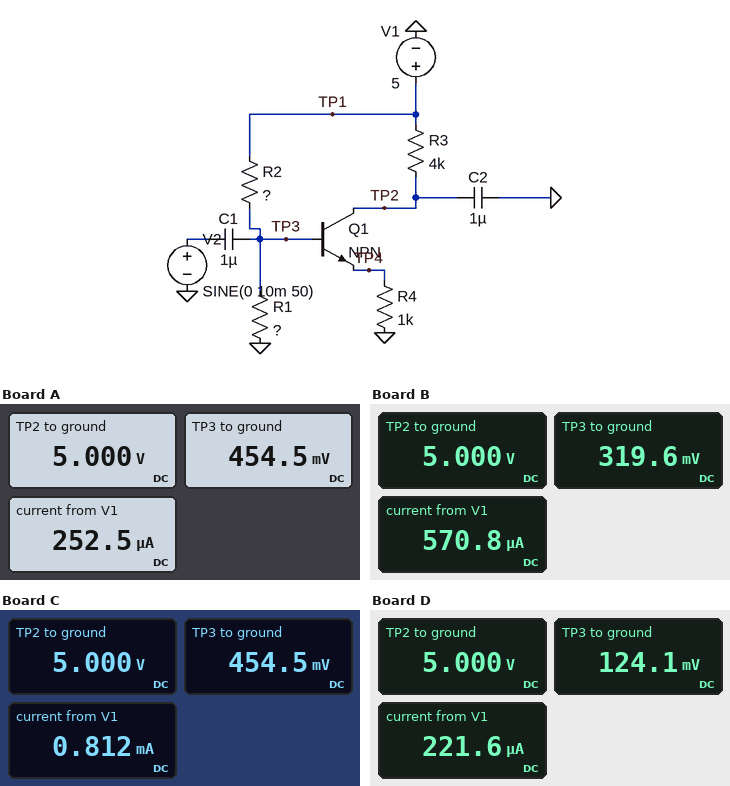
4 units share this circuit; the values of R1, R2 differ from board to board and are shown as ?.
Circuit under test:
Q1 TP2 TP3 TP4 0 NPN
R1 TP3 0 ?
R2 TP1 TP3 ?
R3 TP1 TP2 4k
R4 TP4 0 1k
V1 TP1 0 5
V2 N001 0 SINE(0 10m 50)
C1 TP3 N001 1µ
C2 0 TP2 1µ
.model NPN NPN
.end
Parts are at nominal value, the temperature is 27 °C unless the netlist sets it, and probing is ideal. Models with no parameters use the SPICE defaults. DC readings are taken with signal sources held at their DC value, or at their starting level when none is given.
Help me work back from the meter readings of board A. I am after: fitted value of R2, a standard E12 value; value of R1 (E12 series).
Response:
18 kΩ
1.8 kΩ
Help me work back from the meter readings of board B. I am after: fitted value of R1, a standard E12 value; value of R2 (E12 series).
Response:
560 Ω
8.2 kΩ
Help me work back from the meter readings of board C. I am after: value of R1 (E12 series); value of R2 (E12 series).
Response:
560 Ω
5.6 kΩ
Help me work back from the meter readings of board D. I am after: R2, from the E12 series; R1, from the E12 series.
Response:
22 kΩ
560 Ω
